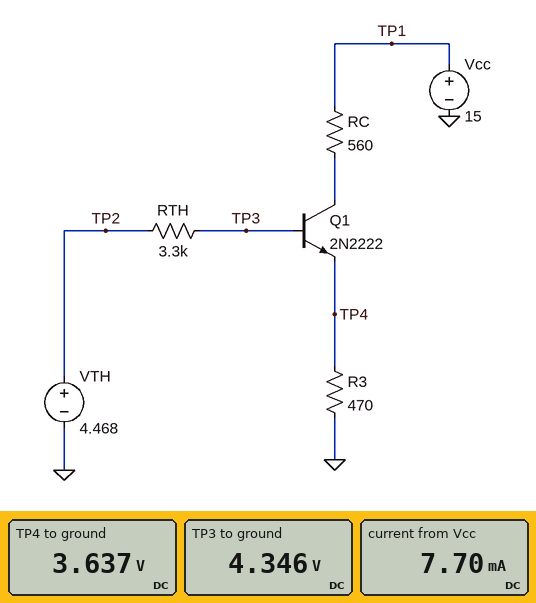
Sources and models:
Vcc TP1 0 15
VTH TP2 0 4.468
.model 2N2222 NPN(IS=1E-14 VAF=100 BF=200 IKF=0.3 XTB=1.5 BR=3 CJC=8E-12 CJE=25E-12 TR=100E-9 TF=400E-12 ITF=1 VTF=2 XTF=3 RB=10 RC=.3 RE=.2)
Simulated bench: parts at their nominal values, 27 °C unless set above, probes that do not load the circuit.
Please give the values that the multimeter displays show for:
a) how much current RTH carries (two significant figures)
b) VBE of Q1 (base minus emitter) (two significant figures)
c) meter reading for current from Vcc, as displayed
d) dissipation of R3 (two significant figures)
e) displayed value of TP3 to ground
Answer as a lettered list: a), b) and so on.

a) 37 µA
b) 710 mV
c) 7.70 mA
d) 28 mW
e) 4.346 V
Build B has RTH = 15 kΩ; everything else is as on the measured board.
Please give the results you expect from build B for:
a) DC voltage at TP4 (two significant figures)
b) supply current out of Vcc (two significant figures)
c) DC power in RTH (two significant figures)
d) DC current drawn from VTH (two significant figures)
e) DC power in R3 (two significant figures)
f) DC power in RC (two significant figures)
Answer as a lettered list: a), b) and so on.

a) 3.3 V
b) 6.9 mA
c) 16 µW
d) 33 µA
e) 23 mW
f) 27 mW
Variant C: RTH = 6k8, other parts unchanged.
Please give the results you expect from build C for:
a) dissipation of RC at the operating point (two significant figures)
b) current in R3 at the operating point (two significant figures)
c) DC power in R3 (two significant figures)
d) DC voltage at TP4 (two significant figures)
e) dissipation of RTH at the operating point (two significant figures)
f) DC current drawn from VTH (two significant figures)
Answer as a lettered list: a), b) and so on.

a) 31 mW
b) 7.5 mA
c) 26 mW
d) 3.5 V
e) 8.7 µW
f) 36 µA
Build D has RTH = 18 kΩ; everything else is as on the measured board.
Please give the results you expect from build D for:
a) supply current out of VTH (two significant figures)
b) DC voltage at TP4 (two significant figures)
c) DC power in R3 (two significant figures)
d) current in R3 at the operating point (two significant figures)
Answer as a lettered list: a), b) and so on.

a) 32 µA
b) 3.2 V
c) 22 mW
d) 6.8 mA
